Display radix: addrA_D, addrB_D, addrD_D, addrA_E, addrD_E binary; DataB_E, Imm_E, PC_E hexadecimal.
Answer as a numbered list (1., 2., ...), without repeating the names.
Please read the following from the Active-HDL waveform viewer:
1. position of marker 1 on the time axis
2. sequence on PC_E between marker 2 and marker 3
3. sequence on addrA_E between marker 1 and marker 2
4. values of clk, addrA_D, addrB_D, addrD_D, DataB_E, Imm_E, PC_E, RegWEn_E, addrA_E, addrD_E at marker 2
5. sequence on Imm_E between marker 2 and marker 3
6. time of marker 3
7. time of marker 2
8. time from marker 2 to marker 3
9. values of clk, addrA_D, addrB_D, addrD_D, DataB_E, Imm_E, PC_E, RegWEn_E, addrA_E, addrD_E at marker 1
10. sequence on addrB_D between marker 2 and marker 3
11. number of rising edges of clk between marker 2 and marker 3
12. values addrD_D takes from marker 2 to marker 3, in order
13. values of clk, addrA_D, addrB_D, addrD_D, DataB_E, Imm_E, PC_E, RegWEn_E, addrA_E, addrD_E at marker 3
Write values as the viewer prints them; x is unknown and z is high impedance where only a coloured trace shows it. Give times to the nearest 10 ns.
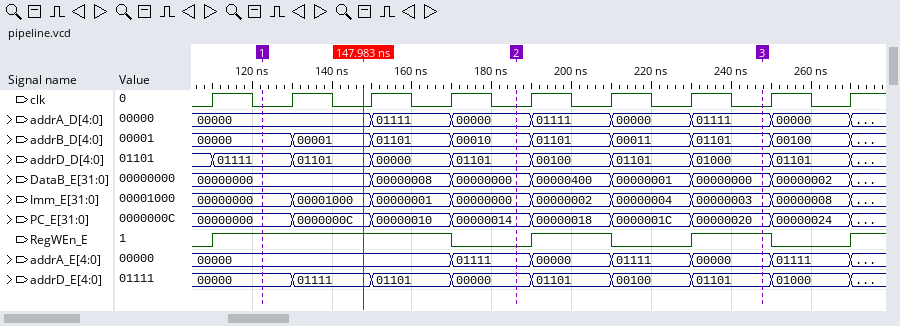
1. 120 ns
2. 00000014, 00000018, 0000001C, 00000020
3. 00000, 01111
4. clk=0, addrA_D=00000, addrB_D=00010, addrD_D=01101, DataB_E=00000000, Imm_E=00000000, PC_E=00000014, RegWEn_E=0, addrA_E=01111, addrD_E=00000
5. 00000000, 00000002, 00000004, 00000003
6. 250 ns
7. 190 ns
8. 60 ns
9. clk=0, addrA_D=00000, addrB_D=00000, addrD_D=01111, DataB_E=00000000, Imm_E=00000000, PC_E=00000000, RegWEn_E=1, addrA_E=00000, addrD_E=00000
10. 00010, 01101, 00011, 01101
11. 3
12. 01101, 00100, 01101, 01000
13. clk=0, addrA_D=01111, addrB_D=01101, addrD_D=01000, DataB_E=00000000, Imm_E=00000003, PC_E=00000020, RegWEn_E=1, addrA_E=00000, addrD_E=01101
